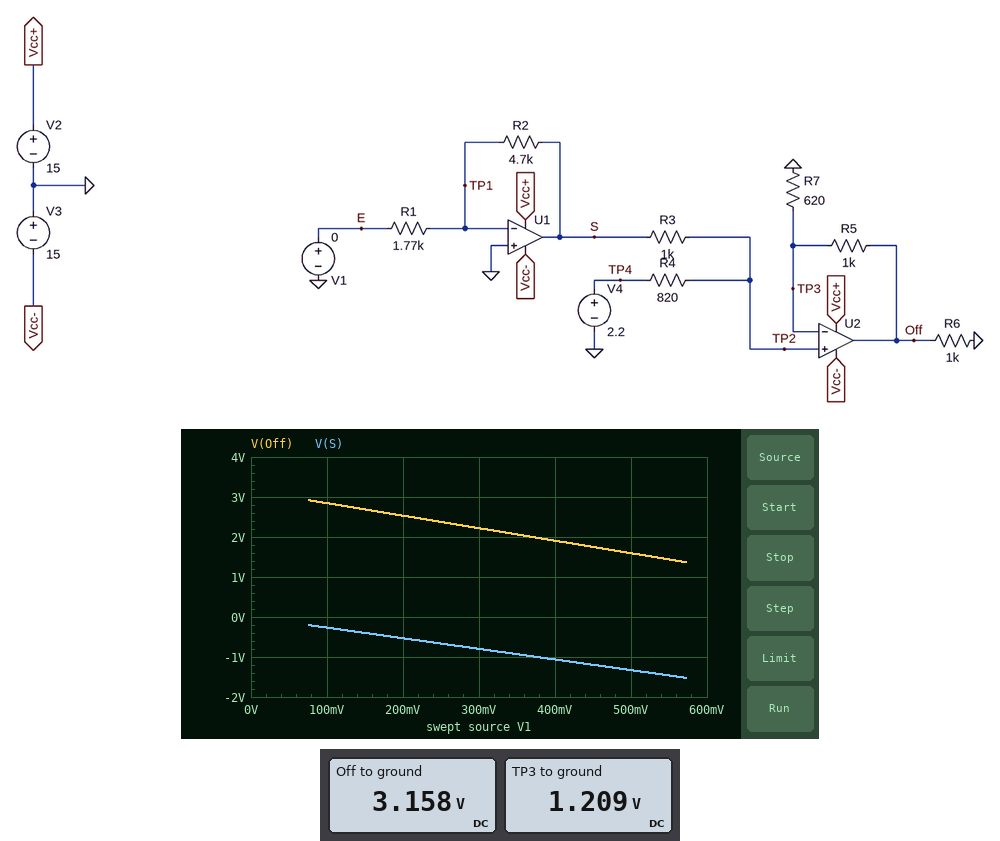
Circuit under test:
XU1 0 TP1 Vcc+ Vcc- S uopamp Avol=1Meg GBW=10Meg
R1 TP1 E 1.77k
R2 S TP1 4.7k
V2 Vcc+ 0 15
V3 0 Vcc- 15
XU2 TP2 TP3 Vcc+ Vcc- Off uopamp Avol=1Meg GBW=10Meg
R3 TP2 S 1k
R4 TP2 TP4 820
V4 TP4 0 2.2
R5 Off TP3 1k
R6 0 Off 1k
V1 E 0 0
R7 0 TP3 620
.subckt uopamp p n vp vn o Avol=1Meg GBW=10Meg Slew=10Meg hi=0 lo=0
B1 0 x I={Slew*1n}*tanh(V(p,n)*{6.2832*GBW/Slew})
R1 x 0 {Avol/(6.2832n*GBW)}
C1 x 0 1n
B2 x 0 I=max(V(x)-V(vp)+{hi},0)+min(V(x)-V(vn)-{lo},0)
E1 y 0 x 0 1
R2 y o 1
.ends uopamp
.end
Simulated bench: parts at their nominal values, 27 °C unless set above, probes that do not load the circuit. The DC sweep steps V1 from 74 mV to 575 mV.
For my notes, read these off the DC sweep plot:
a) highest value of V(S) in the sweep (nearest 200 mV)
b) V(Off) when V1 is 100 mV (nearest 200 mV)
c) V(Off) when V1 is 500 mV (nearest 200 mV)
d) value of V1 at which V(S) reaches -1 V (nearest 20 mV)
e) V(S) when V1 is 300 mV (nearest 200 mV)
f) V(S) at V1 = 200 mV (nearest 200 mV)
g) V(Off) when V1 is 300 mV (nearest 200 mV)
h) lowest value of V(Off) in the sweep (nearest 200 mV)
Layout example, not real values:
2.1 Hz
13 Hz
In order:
-200 mV
2.8 V
1.6 V
380 mV
-800 mV
-600 mV
2.2 V
1.4 V
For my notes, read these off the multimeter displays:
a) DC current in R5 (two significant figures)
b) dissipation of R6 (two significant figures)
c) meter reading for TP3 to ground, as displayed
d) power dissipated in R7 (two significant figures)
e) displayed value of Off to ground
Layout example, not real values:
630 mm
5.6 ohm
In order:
1.9 mA
10 mW
1.209 V
2.4 mW
3.158 V
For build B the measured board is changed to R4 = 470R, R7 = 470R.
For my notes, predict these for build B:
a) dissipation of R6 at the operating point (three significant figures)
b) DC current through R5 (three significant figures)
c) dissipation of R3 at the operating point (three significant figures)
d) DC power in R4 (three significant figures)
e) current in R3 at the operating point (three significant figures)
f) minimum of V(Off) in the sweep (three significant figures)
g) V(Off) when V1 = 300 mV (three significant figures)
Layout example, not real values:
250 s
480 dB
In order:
21.9 mW
3.18 mA
2.24 mW
1.05 mW
1.50 mA
3.15 V
3.88 V
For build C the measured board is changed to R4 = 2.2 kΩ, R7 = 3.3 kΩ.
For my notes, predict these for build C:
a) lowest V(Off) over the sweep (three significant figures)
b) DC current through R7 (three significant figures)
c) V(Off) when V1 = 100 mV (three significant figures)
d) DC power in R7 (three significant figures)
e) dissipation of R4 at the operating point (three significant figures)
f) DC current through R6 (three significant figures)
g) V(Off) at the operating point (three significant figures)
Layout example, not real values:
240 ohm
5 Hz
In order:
-472 mV
208 µA
658 mV
143 µW
1.04 mW
896 µA
896 mV
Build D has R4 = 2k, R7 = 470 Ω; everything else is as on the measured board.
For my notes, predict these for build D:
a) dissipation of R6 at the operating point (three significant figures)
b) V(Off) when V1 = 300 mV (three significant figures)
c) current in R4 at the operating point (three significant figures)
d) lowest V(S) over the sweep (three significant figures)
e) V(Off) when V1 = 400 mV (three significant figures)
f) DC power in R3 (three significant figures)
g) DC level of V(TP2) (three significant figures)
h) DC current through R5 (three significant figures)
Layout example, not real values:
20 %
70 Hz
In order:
5.26 mW
633 mV
733 µA
-1.53 V
78.9 mV
538 µW
733 mV
1.56 mA
